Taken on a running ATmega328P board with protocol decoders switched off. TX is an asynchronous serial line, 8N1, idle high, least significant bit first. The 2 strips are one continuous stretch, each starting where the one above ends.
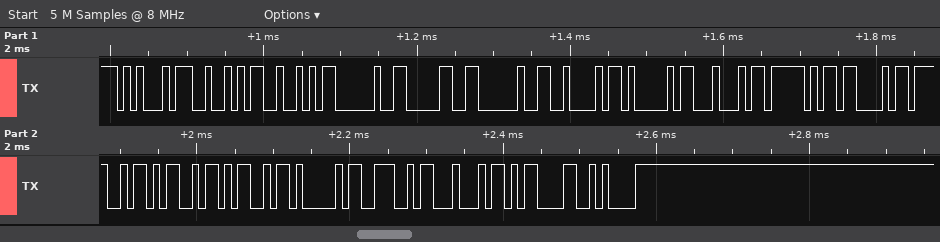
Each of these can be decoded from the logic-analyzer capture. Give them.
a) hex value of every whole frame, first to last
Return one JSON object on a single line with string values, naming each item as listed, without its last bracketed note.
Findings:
{"hex value of every whole frame, first to last": "0x45 0x52 0x52 0x20 0x30 0x20 0x42 0x41 0x44 0x5F 0x43 0x4F 0x4D 0x4D 0x41 0x4E 0x44 0x0D 0x0A"}
